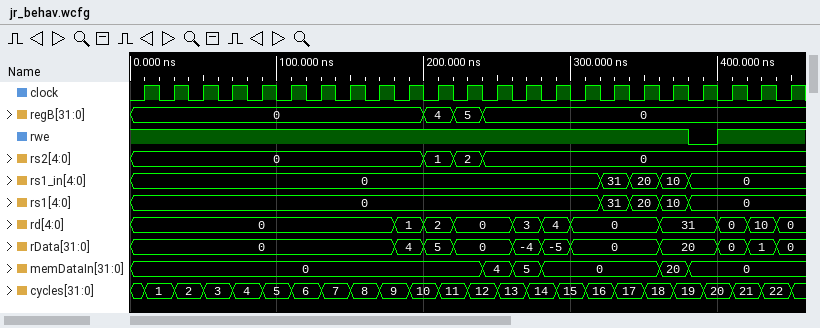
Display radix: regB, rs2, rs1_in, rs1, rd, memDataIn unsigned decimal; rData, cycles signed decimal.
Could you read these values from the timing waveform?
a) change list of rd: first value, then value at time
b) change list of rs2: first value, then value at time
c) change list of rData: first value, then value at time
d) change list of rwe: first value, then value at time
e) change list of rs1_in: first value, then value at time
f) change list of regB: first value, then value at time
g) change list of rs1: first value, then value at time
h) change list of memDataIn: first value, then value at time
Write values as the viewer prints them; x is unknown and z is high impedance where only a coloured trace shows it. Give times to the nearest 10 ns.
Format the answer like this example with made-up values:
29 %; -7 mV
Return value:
0, 1 at 180 ns, 2 at 200 ns, 0 at 220 ns, 3 at 260 ns, 4 at 280 ns, 0 at 300 ns, 31 at 360 ns, 0 at 400 ns, 10 at 420 ns, 0 at 440 ns; 0, 1 at 200 ns, 2 at 220 ns, 0 at 240 ns; 0, 4 at 180 ns, 5 at 200 ns, 0 at 220 ns, -4 at 260 ns, -5 at 280 ns, 0 at 300 ns, 20 at 360 ns, 0 at 400 ns, 1 at 420 ns, 0 at 440 ns; 1, 0 at 380 ns, 1 at 400 ns; 0, 31 at 320 ns, 20 at 340 ns, 10 at 360 ns, 0 at 380 ns; 0, 4 at 200 ns, 5 at 220 ns, 0 at 240 ns; 0, 31 at 320 ns, 20 at 340 ns, 10 at 360 ns, 0 at 380 ns; 0, 4 at 240 ns, 5 at 260 ns, 0 at 280 ns, 20 at 360 ns, 0 at 380 ns
